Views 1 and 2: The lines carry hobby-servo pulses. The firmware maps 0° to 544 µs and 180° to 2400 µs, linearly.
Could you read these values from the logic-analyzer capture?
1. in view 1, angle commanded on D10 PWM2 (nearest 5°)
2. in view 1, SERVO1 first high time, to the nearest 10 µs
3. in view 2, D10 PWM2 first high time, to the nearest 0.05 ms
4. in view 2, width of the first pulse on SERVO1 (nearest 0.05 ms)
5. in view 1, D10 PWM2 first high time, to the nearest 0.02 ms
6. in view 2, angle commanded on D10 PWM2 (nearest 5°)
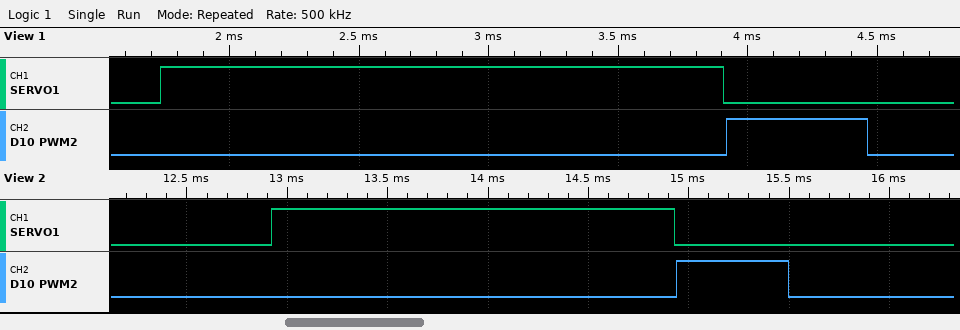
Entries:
0°
2170 µs
0.55 ms
2.00 ms
0.54 ms
0°
